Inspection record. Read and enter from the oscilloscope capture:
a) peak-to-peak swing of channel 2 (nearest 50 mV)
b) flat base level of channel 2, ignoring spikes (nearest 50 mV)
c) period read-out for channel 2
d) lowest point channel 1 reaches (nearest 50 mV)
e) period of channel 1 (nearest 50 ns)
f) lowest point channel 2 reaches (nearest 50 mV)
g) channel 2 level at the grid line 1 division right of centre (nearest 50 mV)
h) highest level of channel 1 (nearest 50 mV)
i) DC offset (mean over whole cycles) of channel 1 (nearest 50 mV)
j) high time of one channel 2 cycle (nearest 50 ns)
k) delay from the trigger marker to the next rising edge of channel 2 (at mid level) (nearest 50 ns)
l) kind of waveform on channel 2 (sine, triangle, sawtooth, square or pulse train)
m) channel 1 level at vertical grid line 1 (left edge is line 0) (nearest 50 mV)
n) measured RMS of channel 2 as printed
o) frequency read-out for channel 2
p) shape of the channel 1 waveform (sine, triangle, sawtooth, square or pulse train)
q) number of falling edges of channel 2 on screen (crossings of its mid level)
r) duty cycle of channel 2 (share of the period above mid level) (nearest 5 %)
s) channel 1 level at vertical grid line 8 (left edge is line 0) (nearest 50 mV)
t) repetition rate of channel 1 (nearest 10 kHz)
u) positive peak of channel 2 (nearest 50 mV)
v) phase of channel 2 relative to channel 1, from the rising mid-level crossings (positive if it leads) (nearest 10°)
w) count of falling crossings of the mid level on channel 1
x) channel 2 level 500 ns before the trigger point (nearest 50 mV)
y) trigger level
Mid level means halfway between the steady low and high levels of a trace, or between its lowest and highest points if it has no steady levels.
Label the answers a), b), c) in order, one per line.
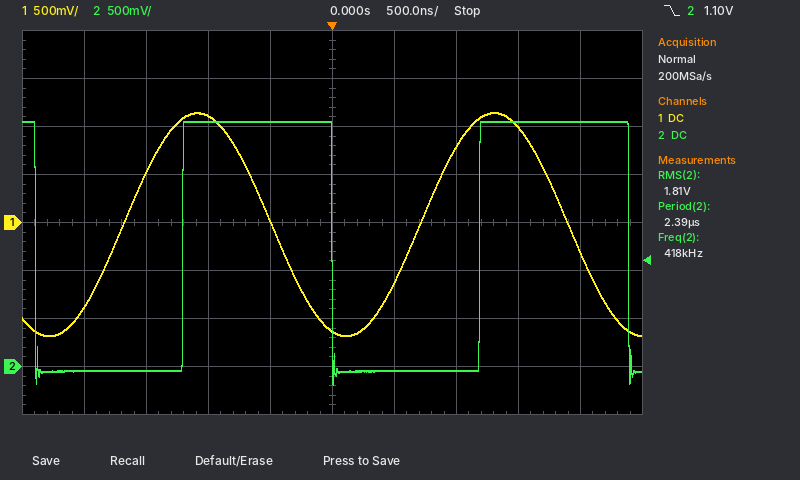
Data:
a) 2.75 V
b) -50 mV
c) 2.39 µs
d) -1.20 V
e) 2.40 µs
f) -200 mV
g) -50 mV
h) 1.15 V
i) 0 mV
j) 1.20 µs
k) 1.20 µs
l) square
m) -900 mV
n) 1.81 V
o) 418 kHz
p) sine
q) 3
r) 50 %
s) 1.00 V
t) 420 kHz
u) 2.55 V
v) -70°
w) 2
x) 2.55 V
y) 1.10 V
